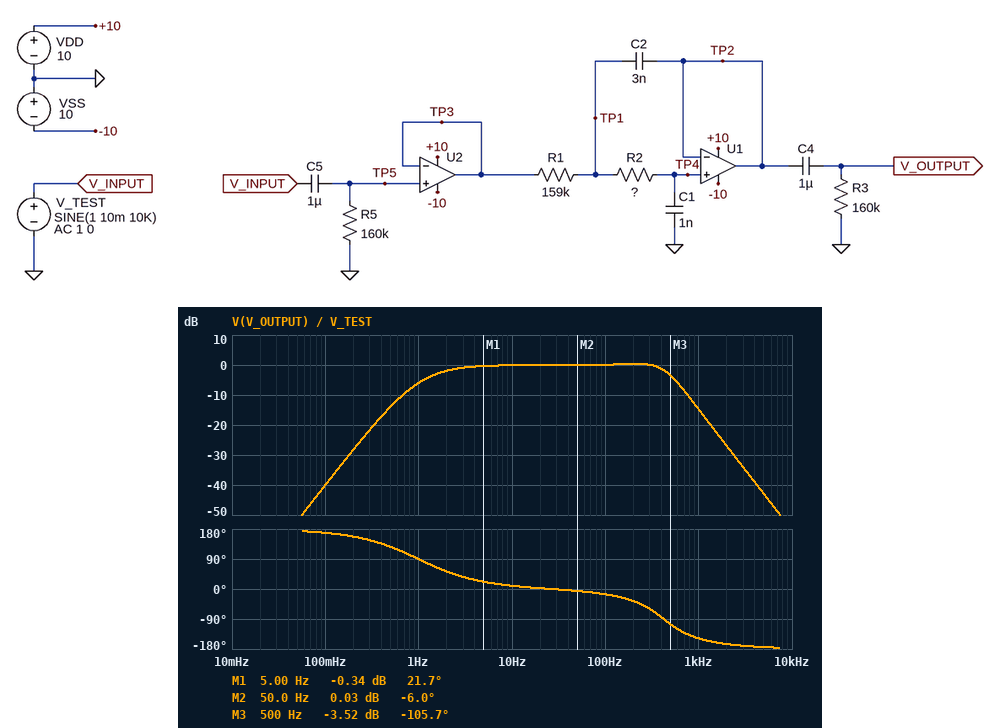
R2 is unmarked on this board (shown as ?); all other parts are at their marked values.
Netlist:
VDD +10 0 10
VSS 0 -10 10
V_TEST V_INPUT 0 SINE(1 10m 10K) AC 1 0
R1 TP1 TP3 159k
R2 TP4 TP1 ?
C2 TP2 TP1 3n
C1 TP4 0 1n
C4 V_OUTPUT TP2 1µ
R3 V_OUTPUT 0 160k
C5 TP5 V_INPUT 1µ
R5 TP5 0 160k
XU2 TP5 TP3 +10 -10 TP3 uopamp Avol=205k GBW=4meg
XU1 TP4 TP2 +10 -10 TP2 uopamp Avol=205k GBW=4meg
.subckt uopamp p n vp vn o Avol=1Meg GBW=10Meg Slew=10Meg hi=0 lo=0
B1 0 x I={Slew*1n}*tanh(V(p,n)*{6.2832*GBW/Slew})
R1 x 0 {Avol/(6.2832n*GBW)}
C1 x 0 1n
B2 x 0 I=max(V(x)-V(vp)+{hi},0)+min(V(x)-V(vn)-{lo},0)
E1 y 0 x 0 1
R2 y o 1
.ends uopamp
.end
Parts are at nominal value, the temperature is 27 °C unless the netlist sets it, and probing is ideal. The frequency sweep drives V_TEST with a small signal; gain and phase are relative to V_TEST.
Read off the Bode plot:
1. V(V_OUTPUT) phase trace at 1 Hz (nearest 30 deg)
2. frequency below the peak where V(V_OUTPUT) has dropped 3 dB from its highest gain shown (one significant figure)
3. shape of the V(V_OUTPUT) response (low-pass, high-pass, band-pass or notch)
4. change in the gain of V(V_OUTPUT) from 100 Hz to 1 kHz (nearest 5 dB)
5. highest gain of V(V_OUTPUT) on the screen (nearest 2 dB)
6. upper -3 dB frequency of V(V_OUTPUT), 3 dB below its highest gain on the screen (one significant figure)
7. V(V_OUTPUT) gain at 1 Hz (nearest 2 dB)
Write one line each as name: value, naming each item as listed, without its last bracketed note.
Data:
V(V_OUTPUT) phase trace at 1 Hz: 90 deg
frequency below the peak where V(V_OUTPUT) has dropped 3 dB from its highest gain shown: 2 Hz
shape of the V(V_OUTPUT) response: band-pass
change in the gain of V(V_OUTPUT) from 100 Hz to 1 kHz: -15 dB
highest gain of V(V_OUTPUT) on the screen: 0 dB
upper -3 dB frequency of V(V_OUTPUT), 3 dB below its highest gain on the screen: 500 Hz
V(V_OUTPUT) gain at 1 Hz: -6 dB
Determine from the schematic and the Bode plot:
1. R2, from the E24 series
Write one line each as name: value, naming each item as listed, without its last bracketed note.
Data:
R2, from the E24 series: 300 kΩ
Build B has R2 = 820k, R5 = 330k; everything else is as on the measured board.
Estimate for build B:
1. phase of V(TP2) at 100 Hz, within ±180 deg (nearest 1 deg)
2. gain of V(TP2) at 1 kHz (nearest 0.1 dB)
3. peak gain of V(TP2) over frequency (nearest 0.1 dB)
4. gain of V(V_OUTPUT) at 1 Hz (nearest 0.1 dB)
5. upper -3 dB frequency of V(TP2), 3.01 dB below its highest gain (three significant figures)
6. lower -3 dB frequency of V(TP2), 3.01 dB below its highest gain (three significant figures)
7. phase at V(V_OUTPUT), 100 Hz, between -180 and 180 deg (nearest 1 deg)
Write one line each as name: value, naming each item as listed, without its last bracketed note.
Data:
phase of V(TP2) at 100 Hz, within ±180 deg: -36 deg
gain of V(TP2) at 1 kHz: -23.9 dB
peak gain of V(TP2) over frequency: 0 dB
gain of V(V_OUTPUT) at 1 Hz: -3.9 dB
upper -3 dB frequency of V(TP2), 3.01 dB below its highest gain: 228 Hz
lower -3 dB frequency of V(TP2), 3.01 dB below its highest gain: 481 mHz
phase at V(V_OUTPUT), 100 Hz, between -180 and 180 deg: -35 deg
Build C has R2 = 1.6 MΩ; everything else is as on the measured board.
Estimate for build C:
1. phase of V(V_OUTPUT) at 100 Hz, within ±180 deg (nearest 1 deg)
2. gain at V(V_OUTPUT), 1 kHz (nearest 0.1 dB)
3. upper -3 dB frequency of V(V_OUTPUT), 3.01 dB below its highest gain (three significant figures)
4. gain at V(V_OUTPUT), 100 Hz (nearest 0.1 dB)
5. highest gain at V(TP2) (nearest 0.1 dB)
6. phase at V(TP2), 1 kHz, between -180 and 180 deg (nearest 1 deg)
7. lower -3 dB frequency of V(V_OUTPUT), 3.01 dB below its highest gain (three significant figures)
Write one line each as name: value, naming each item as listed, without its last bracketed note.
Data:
phase of V(V_OUTPUT) at 100 Hz, within ±180 deg: -57 deg
gain at V(V_OUTPUT), 1 kHz: -29.9 dB
upper -3 dB frequency of V(V_OUTPUT), 3.01 dB below its highest gain: 118 Hz
gain at V(V_OUTPUT), 100 Hz: -2.3 dB
highest gain at V(TP2): -0.1 dB
phase at V(TP2), 1 kHz, between -180 and 180 deg: -159 deg
lower -3 dB frequency of V(V_OUTPUT), 3.01 dB below its highest gain: 1.52 Hz
